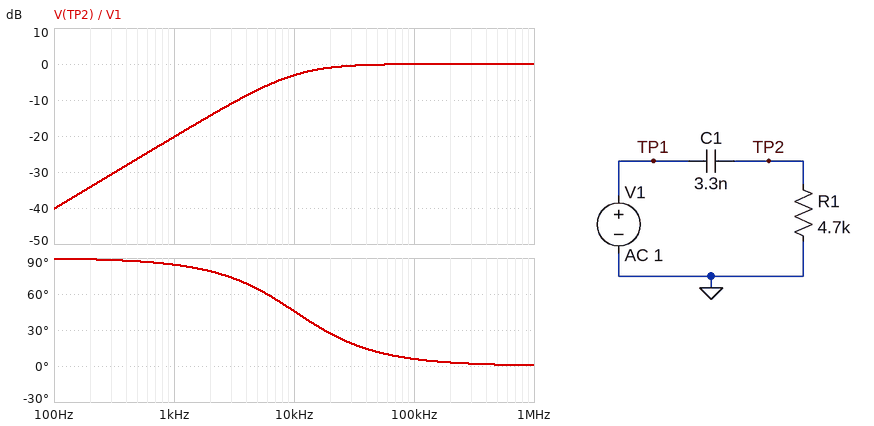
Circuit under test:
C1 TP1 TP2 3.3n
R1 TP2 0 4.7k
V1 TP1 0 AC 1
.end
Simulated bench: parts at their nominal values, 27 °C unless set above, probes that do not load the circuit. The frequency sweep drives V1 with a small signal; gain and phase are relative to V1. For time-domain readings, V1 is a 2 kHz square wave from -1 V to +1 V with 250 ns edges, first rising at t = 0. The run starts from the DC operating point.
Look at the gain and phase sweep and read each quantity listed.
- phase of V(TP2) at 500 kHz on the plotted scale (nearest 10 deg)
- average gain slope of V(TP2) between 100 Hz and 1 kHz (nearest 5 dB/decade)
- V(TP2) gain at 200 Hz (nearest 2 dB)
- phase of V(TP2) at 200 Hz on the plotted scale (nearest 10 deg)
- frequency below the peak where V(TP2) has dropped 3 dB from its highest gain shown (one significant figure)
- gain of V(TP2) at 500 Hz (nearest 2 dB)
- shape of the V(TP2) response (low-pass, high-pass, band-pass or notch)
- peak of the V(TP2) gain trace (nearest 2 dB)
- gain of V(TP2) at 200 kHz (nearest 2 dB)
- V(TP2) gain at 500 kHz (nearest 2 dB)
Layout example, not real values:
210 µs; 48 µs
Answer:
0 deg; 20 dB/decade; -34 dB; 90 deg; 10 kHz; -26 dB; high-pass; 0 dB; 0 dB; 0 dB
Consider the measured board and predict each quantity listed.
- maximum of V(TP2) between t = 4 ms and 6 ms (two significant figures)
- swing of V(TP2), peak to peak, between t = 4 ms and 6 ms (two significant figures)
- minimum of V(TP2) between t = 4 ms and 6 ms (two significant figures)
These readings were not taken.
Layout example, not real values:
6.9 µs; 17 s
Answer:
2.0 V; 4.0 V; -2.0 V
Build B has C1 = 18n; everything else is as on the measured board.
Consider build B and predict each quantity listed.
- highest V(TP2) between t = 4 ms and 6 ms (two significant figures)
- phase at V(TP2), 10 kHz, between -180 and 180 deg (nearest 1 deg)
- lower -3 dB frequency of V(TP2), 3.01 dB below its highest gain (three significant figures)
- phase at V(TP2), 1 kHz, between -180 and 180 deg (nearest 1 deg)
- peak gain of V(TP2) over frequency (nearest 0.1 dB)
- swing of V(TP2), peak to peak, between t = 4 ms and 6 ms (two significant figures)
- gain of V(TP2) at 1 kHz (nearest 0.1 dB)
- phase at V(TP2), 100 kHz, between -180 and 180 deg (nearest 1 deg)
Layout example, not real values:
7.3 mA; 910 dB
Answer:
1.9 V; 11 deg; 1.88 kHz; 62 deg; 0 dB; 3.8 V; -6.6 dB; 1 deg
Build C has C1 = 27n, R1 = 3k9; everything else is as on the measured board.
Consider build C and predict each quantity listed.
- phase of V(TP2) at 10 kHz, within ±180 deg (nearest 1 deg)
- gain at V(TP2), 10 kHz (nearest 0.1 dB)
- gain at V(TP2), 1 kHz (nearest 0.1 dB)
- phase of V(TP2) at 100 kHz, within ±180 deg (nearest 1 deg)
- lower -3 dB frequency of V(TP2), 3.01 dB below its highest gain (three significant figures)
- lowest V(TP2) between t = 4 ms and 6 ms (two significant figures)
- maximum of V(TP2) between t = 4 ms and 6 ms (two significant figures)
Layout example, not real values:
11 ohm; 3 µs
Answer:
9 deg; -0.1 dB; -5.2 dB; 1 deg; 1.51 kHz; -1.8 V; 1.8 V
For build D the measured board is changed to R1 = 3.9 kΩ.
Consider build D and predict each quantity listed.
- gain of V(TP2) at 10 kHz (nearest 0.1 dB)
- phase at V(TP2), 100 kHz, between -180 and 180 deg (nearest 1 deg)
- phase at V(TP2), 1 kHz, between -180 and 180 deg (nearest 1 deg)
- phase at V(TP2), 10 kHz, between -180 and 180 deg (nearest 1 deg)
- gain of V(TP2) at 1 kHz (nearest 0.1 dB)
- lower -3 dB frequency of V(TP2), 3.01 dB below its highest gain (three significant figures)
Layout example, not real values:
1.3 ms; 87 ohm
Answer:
-4.0 dB; 7 deg; 85 deg; 51 deg; -21.9 dB; 12.4 kHz
